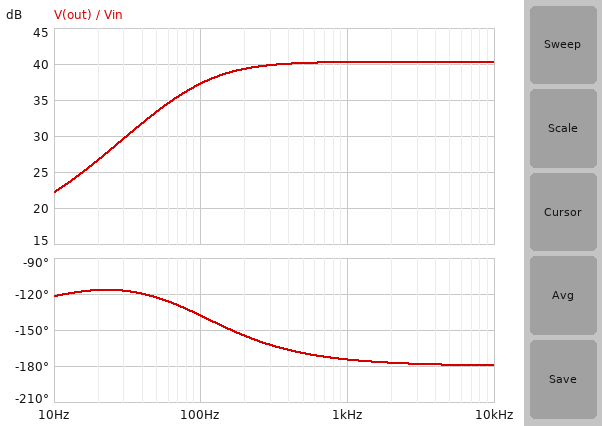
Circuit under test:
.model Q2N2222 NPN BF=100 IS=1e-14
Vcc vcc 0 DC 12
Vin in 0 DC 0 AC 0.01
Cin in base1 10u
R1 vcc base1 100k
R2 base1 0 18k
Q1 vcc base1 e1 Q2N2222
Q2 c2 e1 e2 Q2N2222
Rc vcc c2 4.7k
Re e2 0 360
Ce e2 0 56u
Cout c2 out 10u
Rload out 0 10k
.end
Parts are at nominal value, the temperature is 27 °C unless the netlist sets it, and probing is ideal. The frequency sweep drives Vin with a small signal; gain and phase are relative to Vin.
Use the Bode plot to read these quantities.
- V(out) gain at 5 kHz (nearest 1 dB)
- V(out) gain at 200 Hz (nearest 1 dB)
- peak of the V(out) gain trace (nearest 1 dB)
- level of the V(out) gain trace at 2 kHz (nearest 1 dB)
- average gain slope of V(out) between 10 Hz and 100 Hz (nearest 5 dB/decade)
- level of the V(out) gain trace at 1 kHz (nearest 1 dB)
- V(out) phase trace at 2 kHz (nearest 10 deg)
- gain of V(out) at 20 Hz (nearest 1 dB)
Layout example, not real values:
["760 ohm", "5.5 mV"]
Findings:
["40 dB", "39 dB", "40 dB", "40 dB", "15 dB/decade", "40 dB", "-180 deg", "27 dB"]
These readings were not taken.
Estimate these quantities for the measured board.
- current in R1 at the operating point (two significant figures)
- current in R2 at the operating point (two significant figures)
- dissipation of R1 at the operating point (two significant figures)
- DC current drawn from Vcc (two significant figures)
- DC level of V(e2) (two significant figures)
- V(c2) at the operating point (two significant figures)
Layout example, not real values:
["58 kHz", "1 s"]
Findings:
["100 µA", "100 µA", "1.0 mW", "1.8 mA", "610 mV", "4.1 V"]
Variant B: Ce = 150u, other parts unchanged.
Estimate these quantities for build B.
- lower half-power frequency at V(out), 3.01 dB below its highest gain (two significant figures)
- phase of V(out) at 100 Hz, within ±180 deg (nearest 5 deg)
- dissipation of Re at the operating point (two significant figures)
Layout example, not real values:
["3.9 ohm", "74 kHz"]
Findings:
["38 Hz", "-160 deg", "1.0 mW"]
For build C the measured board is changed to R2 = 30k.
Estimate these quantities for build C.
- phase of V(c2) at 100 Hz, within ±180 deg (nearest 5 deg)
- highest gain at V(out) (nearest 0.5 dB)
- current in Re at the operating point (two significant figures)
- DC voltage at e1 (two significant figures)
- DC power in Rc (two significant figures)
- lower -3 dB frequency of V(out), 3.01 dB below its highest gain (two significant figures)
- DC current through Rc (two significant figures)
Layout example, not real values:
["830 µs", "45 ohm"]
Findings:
["-75 deg", "-2.0 dB", "3.3 mA", "1.9 V", "25 mW", "2.0 Hz", "2.3 mA"]
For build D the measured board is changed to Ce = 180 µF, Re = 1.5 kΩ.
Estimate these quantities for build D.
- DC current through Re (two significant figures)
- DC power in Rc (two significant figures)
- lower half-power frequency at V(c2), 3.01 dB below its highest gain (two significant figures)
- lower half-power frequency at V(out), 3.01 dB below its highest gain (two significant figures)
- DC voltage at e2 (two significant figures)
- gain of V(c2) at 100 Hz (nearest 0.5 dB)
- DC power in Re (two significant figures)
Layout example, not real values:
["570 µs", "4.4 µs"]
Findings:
["450 µA", "950 µW", "8.3 Hz", "8.6 Hz", "680 mV", "29.0 dB", "310 µW"]
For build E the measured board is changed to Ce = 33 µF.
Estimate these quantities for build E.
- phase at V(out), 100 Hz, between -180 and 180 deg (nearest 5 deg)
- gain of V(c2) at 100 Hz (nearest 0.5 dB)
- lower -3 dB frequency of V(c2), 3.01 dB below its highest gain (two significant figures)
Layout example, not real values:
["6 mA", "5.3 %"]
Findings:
["-125 deg", "34.5 dB", "170 Hz"]
